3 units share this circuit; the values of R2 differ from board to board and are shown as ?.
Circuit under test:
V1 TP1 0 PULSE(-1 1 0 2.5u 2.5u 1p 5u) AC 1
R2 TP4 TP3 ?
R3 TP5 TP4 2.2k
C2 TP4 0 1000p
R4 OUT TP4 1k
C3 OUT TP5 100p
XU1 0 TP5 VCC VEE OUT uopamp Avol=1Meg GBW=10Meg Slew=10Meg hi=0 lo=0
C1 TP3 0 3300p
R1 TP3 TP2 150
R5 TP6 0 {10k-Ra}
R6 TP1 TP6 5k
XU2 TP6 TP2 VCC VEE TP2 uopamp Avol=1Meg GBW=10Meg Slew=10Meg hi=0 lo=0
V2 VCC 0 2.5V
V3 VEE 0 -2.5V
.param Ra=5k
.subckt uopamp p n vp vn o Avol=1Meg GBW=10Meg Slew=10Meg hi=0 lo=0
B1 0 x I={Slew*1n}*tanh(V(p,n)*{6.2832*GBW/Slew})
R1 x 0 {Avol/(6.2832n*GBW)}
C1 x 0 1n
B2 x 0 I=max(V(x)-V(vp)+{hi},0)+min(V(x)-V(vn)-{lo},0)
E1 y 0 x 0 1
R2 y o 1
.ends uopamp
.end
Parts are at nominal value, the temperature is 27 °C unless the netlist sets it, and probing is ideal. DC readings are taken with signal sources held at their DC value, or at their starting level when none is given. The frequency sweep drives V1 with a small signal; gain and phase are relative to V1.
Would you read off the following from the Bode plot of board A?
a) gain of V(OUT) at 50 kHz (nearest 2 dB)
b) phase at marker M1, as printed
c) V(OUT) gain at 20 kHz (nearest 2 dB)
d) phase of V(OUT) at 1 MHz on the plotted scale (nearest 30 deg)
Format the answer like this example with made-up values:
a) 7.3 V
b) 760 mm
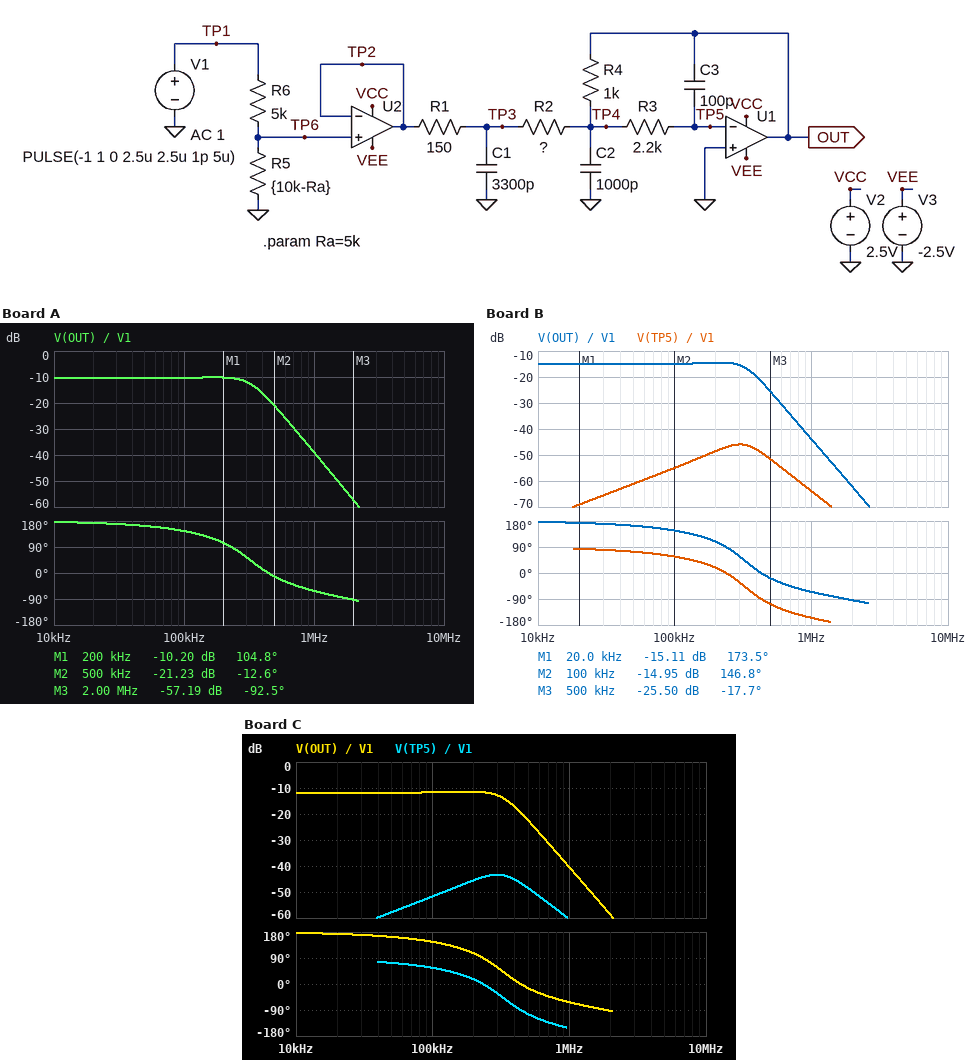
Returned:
a) -10 dB
b) 104.8 deg
c) -10 dB
d) -60 deg
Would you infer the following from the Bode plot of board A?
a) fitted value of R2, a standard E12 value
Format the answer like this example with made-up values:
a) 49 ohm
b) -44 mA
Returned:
a) 1.5 kΩ
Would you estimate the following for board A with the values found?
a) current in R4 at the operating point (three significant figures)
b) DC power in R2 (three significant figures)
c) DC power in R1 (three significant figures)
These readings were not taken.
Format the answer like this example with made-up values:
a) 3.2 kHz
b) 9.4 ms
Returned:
a) 303 µA
b) 138 µW
c) 13.8 µW
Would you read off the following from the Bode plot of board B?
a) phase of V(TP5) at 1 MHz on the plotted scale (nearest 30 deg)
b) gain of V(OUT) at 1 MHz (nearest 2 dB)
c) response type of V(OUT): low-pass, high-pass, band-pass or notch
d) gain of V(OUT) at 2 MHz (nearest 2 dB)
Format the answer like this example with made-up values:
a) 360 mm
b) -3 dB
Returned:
a) -150 deg
b) -44 dB
c) low-pass
d) -62 dB
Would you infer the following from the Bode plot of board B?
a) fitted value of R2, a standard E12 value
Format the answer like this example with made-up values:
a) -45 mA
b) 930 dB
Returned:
a) 2.7 kΩ
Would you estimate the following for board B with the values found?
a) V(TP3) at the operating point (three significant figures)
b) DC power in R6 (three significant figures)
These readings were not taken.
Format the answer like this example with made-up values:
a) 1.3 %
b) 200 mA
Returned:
a) -474 mV
b) 50.0 µW
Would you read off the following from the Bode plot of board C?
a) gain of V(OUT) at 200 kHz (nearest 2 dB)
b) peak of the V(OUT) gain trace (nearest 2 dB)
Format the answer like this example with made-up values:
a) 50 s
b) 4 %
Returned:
a) -12 dB
b) -12 dB
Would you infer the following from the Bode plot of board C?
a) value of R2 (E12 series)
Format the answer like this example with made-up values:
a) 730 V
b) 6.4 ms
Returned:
a) 1.8 kΩ
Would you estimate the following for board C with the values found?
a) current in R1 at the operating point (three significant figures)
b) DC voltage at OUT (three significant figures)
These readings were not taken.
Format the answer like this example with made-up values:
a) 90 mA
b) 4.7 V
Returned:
a) 256 µA
b) 256 mV
